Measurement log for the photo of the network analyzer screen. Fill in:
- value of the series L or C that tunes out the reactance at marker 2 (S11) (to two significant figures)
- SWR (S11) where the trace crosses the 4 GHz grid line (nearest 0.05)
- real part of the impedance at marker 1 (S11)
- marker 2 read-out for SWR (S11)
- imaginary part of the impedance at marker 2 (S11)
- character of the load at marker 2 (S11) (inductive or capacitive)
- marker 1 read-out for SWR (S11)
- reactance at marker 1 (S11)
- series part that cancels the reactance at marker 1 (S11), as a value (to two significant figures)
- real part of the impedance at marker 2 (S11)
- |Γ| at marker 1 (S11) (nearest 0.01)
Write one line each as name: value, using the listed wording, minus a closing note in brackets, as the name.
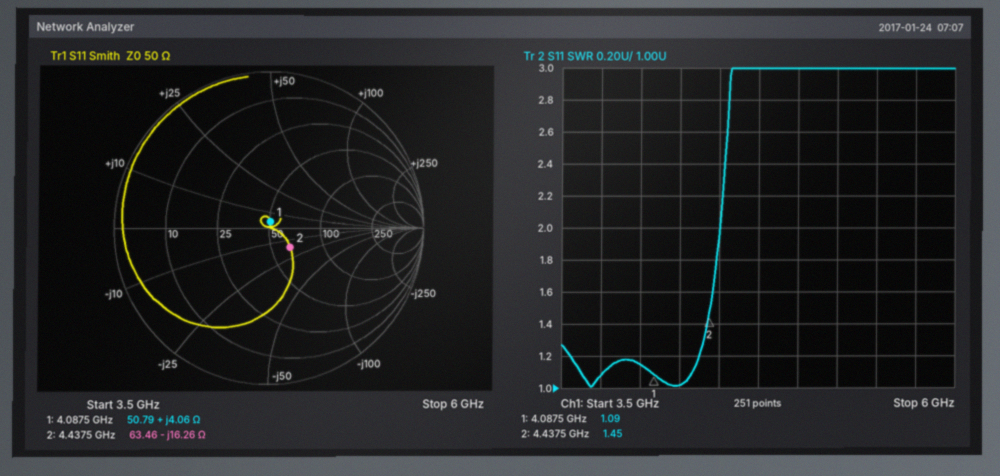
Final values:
value of the series L or C that tunes out the reactance at marker 2 (S11): 580 pH
SWR (S11) where the trace crosses the 4 GHz grid line: 1.15
real part of the impedance at marker 1: 50.79 Ω
marker 2 read-out for SWR: 1.45
imaginary part of the impedance at marker 2: -16.26 Ω
character of the load at marker 2 (S11): capacitive
marker 1 read-out for SWR: 1.09
reactance at marker 1: +4.06 Ω
series part that cancels the reactance at marker 1 (S11), as a value: 9.6 pF
real part of the impedance at marker 2: 63.46 Ω
|Γ| at marker 1 (S11): 0.04
